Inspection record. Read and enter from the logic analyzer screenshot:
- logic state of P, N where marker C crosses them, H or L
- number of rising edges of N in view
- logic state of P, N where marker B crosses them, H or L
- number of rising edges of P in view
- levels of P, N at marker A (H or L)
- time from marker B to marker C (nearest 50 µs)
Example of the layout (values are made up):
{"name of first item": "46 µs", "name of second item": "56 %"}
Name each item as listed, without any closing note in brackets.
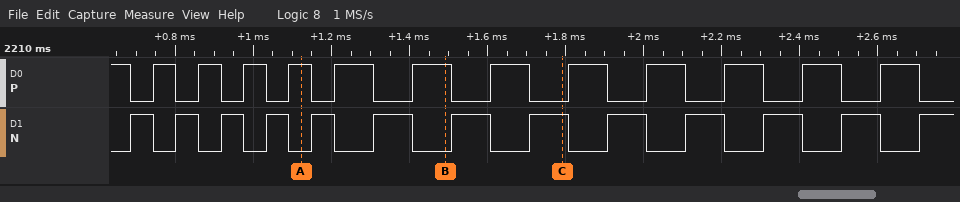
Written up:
{"logic state of P, N where marker C crosses them, H or L": "P=L, N=H", "number of rising edges of N in view": "13", "logic state of P, N where marker B crosses them, H or L": "P=H, N=L", "number of rising edges of P in view": "12", "levels of P, N at marker A": "P=H, N=L", "time from marker B to marker C": "300 µs"}
